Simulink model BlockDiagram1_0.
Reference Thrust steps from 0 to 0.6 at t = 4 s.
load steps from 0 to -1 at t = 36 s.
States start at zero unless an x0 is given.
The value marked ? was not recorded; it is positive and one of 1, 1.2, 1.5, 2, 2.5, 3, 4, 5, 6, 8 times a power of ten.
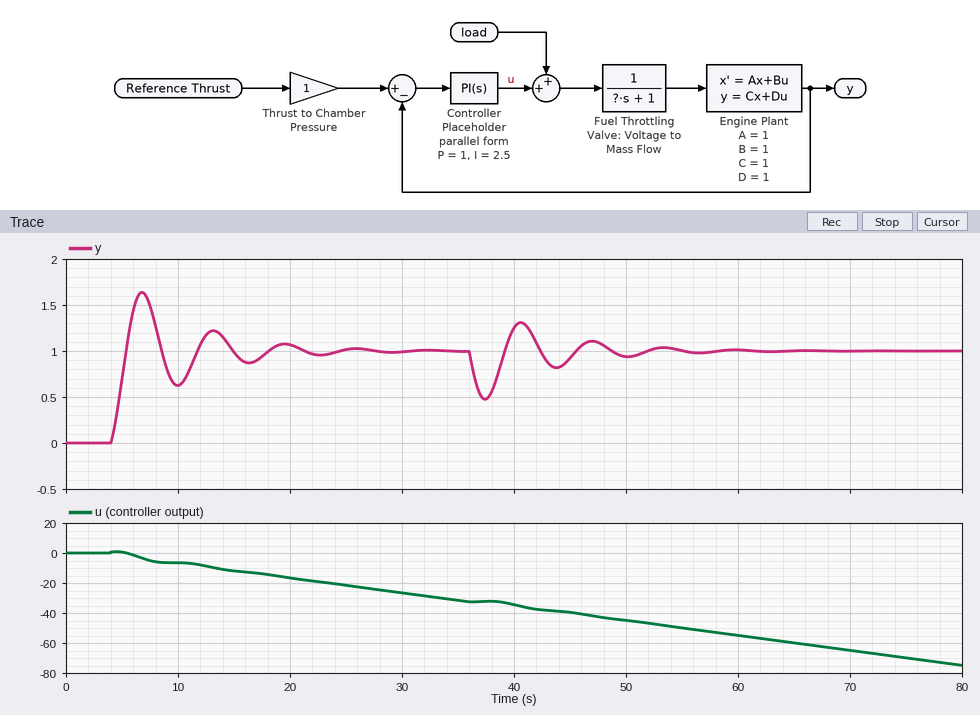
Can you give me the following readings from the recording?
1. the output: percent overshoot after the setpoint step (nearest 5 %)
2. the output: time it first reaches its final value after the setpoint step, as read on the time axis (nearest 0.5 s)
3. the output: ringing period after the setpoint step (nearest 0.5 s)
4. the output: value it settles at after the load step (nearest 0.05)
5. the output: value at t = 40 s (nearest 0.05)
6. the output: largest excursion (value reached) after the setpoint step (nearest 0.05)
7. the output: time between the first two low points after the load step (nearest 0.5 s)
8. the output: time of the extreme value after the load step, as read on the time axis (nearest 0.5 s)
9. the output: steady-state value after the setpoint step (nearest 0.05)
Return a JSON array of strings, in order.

["65 %", "5.5 s", "6.5 s", "1.00", "1.25", "1.65", "6.5 s", "37.5 s", "1.00"]
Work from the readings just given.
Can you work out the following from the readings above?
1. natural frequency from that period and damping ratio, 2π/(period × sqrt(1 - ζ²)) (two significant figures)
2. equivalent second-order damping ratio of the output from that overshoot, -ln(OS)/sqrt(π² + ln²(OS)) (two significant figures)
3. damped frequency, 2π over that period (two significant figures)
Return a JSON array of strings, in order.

["0.98 rad/s", "0.14", "0.97 rad/s"]
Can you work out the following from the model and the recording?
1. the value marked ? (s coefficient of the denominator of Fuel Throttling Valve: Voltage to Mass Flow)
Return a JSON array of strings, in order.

["1.5"]
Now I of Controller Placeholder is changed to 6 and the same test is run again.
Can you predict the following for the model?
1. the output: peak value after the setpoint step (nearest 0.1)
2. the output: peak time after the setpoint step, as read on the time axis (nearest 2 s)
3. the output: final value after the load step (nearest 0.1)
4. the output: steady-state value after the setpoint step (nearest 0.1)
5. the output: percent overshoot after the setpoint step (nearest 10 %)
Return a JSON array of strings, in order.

["1.3", "6 s", "0.7", "0.7", "80 %"]
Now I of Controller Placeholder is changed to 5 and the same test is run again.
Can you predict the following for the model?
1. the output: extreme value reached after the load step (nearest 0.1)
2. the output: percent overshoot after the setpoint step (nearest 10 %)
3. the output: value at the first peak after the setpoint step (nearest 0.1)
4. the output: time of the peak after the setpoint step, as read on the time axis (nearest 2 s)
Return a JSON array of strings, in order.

["0.4", "80 %", "1.3", "6 s"]
